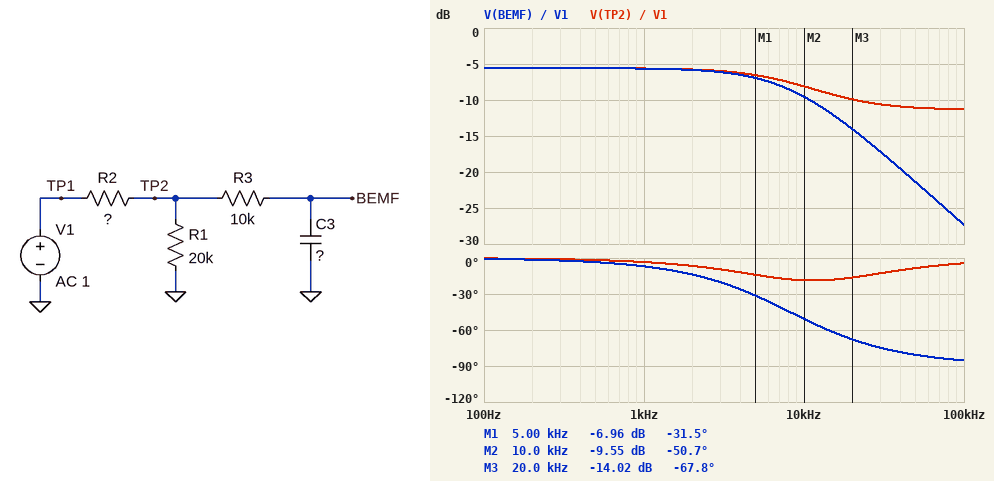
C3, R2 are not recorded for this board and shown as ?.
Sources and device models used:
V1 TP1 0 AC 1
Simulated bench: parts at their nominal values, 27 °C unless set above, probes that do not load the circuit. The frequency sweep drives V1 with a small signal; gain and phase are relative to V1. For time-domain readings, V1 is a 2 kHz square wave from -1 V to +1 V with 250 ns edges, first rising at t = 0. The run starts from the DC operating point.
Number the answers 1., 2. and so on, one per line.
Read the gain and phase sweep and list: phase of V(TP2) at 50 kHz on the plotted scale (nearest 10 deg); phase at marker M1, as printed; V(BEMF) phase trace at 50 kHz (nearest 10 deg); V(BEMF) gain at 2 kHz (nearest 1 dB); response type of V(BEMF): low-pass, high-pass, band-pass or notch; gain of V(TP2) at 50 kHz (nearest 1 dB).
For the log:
1. -10 deg
2. -31.5 deg
3. -80 deg
4. -6 dB
5. low-pass
6. -11 dB
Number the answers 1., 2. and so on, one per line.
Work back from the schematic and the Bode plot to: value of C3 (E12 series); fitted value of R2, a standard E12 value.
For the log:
1. 1 nF
2. 18 kΩ
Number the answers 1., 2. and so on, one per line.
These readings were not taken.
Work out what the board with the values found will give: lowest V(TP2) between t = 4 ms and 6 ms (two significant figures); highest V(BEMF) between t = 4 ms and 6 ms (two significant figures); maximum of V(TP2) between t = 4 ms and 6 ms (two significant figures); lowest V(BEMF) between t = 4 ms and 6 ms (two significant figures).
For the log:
1. -530 mV
2. 530 mV
3. 530 mV
4. -530 mV
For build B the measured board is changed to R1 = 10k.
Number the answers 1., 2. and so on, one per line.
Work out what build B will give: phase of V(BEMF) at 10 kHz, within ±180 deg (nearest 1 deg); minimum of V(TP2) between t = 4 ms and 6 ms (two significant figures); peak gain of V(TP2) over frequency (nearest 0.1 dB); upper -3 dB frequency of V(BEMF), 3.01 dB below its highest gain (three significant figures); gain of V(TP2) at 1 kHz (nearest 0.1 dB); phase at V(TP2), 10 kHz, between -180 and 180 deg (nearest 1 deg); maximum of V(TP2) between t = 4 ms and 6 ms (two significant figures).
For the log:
1. -46 deg
2. -360 mV
3. -8.9 dB
4. 9.69 kHz
5. -9.0 dB
6. -14 deg
7. 360 mV
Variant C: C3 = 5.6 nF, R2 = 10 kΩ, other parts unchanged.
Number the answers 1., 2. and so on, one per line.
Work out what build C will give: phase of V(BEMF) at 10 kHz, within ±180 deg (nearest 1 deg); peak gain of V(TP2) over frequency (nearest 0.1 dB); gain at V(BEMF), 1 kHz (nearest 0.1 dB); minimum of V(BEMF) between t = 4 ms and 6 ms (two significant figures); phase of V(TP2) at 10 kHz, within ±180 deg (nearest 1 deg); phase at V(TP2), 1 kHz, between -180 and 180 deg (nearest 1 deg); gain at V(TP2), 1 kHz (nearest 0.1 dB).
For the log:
1. -80 deg
2. -3.5 dB
3. -4.8 dB
4. -580 mV
5. -6 deg
6. -11 deg
7. -4.3 dB
